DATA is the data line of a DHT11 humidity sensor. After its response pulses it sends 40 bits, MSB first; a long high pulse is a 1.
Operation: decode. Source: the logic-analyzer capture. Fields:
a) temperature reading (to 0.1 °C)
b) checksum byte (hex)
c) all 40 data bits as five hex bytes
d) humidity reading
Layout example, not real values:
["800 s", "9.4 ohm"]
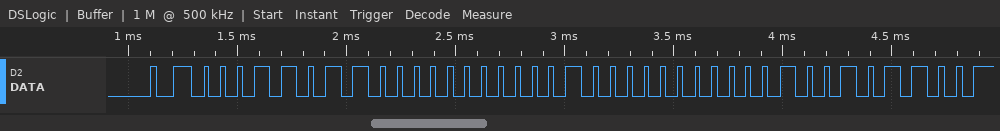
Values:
["16.1 °C", "0x2C", "1B 00 10 01 2C", "27 %"]
